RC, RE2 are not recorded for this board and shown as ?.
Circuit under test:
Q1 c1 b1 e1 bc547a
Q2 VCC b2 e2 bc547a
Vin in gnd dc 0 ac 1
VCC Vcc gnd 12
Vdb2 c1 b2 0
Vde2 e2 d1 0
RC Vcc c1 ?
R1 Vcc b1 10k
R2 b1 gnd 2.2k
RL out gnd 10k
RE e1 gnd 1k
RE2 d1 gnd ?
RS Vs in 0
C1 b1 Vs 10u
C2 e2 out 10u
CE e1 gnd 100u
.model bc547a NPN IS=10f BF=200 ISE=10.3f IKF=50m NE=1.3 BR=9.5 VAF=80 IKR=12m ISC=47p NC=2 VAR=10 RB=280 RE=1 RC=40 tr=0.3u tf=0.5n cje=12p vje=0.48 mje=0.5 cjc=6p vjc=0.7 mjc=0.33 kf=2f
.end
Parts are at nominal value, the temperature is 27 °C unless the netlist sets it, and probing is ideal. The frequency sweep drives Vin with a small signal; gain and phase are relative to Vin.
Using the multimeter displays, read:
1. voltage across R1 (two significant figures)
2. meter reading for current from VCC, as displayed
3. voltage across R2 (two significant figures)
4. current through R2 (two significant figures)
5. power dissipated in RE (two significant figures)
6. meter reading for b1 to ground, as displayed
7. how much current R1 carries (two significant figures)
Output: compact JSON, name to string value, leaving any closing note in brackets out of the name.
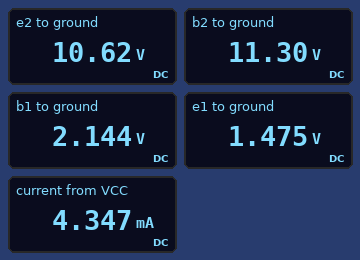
{"voltage across R1": "9.9 V", "meter reading for current from VCC, as displayed": "4.347 mA", "voltage across R2": "2.1 V", "current through R2": "970 µA", "power dissipated in RE": "2.2 mW", "meter reading for b1 to ground, as displayed": "2.144 V", "how much current R1 carries": "990 µA"}
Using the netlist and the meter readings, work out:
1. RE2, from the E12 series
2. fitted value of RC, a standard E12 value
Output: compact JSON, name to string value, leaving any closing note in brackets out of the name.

{"RE2, from the E12 series": "5.6 kΩ", "fitted value of RC, a standard E12 value": "470 Ω"}
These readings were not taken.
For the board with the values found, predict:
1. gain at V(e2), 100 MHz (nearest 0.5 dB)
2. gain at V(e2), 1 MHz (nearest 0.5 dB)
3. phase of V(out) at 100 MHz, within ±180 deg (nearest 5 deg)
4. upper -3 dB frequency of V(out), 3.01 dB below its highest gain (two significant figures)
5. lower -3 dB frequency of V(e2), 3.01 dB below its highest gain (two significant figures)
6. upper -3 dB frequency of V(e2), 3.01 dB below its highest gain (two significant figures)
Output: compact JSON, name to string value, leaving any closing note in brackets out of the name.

{"gain at V(e2), 100 MHz": "-6.5 dB", "gain at V(e2), 1 MHz": "26.5 dB", "phase of V(out) at 100 MHz, within ±180 deg": "25 deg", "upper -3 dB frequency of V(out), 3.01 dB below its highest gain": "4.7 MHz", "lower -3 dB frequency of V(e2), 3.01 dB below its highest gain": "83 Hz", "upper -3 dB frequency of V(e2), 3.01 dB below its highest gain": "4.7 MHz"}
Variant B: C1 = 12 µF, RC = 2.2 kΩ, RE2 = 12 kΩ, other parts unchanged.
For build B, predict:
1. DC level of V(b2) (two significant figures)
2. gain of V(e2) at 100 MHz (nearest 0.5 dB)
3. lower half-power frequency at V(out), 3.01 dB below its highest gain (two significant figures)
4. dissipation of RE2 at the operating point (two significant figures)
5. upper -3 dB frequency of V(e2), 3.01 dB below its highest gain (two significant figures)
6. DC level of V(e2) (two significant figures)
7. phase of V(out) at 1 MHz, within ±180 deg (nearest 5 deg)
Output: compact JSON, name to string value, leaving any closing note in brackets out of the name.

{"DC level of V(b2)": "8.8 V", "gain of V(e2) at 100 MHz": "-2.5 dB", "lower half-power frequency at V(out), 3.01 dB below its highest gain": "80 Hz", "dissipation of RE2 at the operating point": "5.5 mW", "upper -3 dB frequency of V(e2), 3.01 dB below its highest gain": "1.5 MHz", "DC level of V(e2)": "8.1 V", "phase of V(out) at 1 MHz, within ±180 deg": "145 deg"}
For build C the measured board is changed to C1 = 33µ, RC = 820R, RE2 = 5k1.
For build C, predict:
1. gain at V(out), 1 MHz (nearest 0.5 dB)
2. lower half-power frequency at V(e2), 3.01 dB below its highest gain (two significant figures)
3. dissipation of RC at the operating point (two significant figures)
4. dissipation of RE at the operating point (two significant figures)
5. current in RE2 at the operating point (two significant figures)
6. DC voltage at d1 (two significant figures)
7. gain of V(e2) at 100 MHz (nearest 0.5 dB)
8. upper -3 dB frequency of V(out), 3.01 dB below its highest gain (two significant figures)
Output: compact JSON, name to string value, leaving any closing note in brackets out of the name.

{"gain at V(out), 1 MHz": "31.0 dB", "lower half-power frequency at V(e2), 3.01 dB below its highest gain": "78 Hz", "dissipation of RC at the operating point": "1.8 mW", "dissipation of RE at the operating point": "2.2 mW", "current in RE2 at the operating point": "2.0 mA", "DC voltage at d1": "10 V", "gain of V(e2) at 100 MHz": "-4.5 dB", "upper -3 dB frequency of V(out), 3.01 dB below its highest gain": "3.3 MHz"}
